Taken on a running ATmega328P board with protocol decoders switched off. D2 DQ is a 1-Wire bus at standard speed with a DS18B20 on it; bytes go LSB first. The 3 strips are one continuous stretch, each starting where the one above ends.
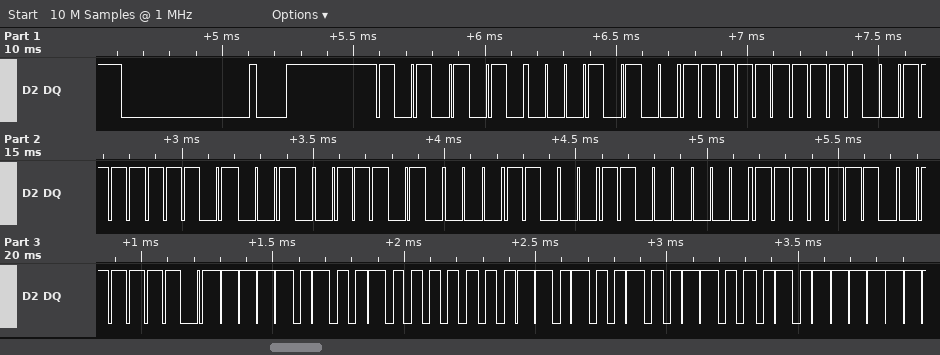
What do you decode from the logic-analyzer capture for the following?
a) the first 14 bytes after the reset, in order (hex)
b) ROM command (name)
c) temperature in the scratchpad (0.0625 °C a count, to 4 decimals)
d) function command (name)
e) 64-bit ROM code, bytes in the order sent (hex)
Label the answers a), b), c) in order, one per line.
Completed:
a) 55 28 FF F3 97 5C 18 03 7F BE 2F 01 4B 46
b) Match ROM
c) 18.9375 °C
d) Read Scratchpad
e) 28 FF F3 97 5C 18 03 7F
